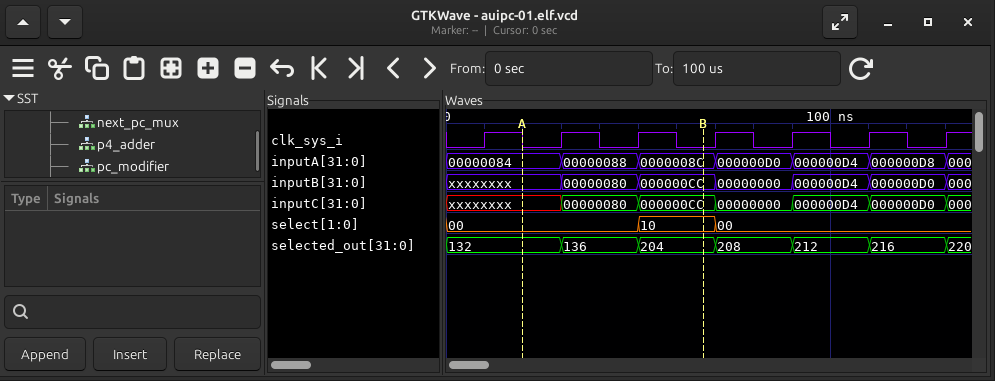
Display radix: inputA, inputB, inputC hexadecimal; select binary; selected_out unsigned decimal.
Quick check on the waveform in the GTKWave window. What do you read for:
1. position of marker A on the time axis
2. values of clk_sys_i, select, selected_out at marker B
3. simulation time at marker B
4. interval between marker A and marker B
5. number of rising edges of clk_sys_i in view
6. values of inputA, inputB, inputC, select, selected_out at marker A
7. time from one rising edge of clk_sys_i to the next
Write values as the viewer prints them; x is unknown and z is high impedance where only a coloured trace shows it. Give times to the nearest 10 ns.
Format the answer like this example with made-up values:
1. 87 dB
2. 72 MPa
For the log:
1. 20 ns
2. clk_sys_i=0, select=10, selected_out=204
3. 70 ns
4. 50 ns
5. 7
6. inputA=00000084, inputB=xxxxxxxx, inputC=xxxxxxxx, select=00, selected_out=132
7. 20 ns
